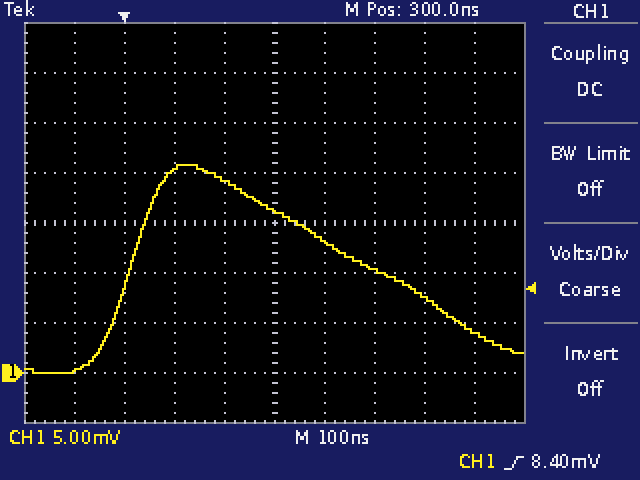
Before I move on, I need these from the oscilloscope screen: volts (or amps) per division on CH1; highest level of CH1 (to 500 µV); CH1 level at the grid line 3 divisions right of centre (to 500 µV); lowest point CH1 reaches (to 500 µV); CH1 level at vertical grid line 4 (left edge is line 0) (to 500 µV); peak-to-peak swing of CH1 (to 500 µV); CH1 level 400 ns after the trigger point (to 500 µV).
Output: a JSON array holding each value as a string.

["5 mV", "21.0 mV", "7.5 mV", "0.0 mV", "19.5 mV", "21.0 mV", "13.0 mV"]
